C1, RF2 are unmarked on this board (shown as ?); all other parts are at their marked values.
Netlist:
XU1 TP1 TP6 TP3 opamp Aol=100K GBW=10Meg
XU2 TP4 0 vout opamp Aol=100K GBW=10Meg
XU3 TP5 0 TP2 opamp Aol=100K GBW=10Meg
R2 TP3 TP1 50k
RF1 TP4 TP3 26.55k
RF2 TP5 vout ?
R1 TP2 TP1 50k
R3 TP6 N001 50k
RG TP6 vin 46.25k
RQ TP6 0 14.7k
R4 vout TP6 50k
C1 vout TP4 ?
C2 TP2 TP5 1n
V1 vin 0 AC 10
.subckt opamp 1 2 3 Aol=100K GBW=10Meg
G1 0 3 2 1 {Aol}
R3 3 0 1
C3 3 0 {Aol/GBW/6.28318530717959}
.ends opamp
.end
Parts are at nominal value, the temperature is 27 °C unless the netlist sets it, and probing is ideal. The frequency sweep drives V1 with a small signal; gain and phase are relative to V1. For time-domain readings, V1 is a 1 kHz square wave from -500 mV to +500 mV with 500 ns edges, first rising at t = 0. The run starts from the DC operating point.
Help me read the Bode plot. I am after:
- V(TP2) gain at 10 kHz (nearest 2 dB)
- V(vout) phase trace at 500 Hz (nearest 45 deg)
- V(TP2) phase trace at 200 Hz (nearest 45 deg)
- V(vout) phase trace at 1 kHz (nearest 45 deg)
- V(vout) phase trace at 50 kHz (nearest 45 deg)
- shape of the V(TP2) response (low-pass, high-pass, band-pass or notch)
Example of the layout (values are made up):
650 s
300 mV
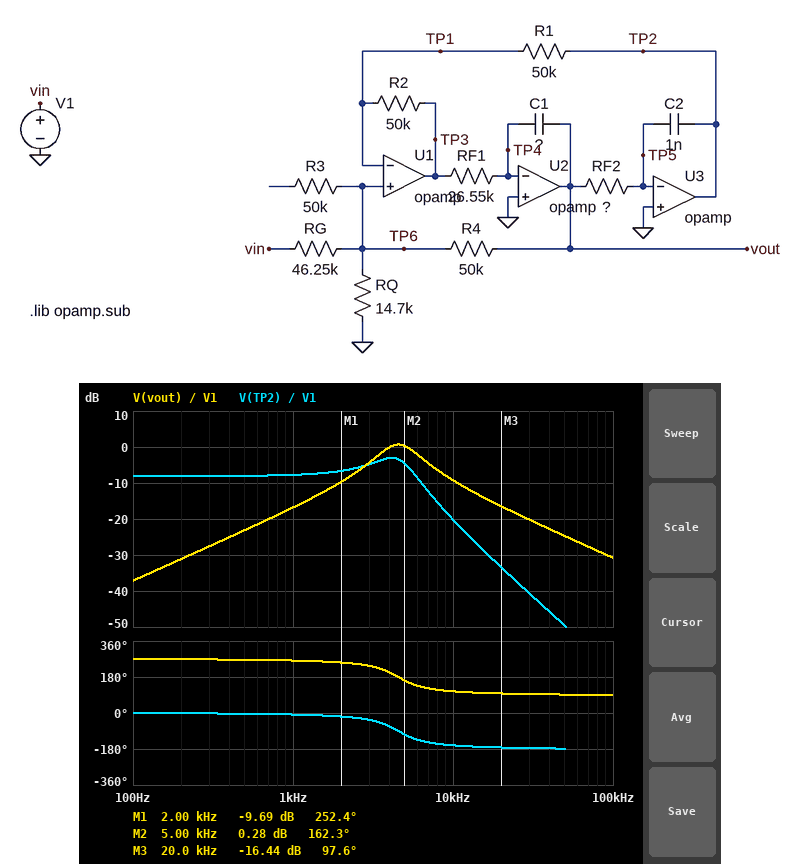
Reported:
-20 dB
270 deg
0 deg
270 deg
90 deg
low-pass
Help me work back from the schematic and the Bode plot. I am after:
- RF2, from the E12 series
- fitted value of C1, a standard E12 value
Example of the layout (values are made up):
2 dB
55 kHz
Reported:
56 kΩ
820 pF
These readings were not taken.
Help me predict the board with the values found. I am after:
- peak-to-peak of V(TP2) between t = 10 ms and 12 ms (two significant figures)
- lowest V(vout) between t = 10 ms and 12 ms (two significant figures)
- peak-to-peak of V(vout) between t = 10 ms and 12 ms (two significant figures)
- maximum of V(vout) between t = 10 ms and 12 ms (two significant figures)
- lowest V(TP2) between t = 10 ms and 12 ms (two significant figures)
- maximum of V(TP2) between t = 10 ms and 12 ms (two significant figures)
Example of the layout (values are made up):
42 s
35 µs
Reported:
690 mV
-420 mV
850 mV
420 mV
-350 mV
350 mV
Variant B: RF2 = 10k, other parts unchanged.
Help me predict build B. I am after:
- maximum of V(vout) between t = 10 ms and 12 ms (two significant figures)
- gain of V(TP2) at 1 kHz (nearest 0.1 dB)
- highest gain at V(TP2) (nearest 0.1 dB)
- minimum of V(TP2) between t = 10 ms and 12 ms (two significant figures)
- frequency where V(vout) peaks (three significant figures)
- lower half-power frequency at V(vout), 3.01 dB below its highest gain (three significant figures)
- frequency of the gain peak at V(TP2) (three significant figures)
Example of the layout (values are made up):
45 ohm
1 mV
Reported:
230 mV
-8.0 dB
4.3 dB
-470 mV
10.8 kHz
9.55 kHz
10.6 kHz
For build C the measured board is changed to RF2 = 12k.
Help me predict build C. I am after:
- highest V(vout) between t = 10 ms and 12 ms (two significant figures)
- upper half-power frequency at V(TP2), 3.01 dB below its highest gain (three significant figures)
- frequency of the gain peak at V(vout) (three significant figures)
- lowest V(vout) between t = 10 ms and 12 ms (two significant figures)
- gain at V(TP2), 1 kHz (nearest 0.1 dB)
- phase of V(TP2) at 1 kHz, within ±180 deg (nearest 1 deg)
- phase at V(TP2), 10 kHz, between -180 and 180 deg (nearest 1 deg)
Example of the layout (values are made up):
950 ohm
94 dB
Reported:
240 mV
10.9 kHz
9.84 kHz
-240 mV
-8.0 dB
-2 deg
-97 deg
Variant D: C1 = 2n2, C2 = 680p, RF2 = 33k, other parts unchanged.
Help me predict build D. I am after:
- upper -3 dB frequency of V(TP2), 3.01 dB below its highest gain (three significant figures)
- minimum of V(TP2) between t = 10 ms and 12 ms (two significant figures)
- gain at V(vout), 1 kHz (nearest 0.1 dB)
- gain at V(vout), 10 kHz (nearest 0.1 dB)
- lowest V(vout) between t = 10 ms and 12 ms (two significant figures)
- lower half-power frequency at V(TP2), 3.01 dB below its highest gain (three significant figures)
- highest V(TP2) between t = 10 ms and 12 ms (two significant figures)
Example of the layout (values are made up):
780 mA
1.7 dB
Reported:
4.81 kHz
-440 mV
-24.6 dB
-17.6 dB
-180 mV
3.81 kHz
440 mV
